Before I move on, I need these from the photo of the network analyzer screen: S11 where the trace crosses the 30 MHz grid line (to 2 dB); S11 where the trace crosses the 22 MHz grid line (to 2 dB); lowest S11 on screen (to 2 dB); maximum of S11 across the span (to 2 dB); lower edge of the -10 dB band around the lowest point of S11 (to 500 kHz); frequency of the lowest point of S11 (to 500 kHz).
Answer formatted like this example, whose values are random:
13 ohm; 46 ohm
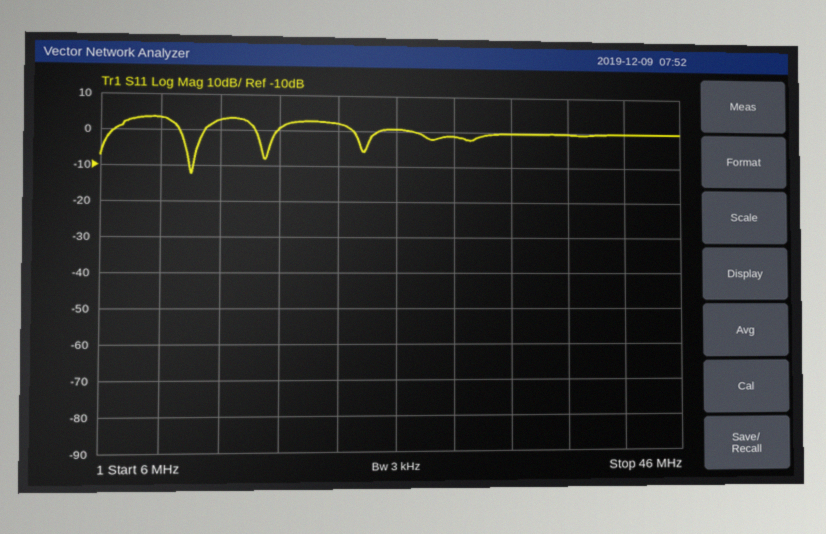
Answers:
-2 dB; 2 dB; -12 dB; 4 dB; 12.0 MHz; 12.0 MHz
